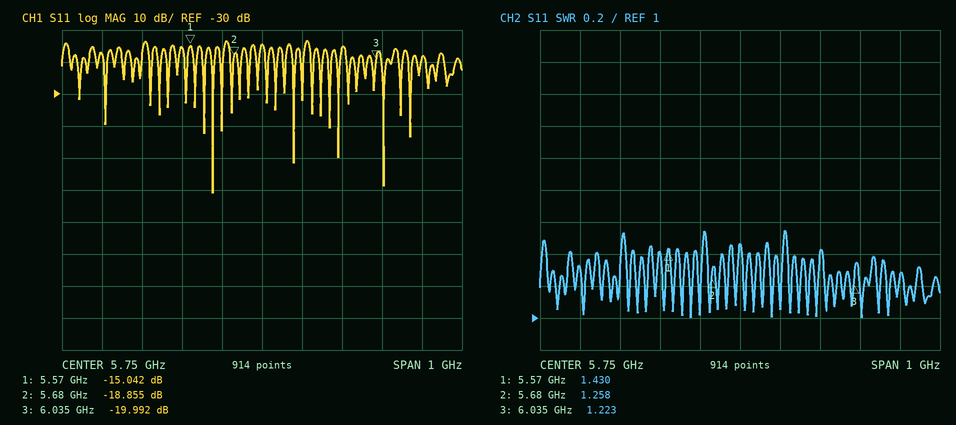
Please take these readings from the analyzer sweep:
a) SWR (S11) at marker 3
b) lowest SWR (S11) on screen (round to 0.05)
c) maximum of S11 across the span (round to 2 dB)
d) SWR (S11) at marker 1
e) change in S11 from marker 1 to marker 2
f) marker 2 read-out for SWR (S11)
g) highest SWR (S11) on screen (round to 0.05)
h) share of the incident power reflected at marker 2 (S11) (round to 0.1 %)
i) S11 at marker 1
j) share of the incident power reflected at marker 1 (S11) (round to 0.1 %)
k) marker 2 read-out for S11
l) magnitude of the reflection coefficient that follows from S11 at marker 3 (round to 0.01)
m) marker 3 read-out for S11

1.223
1.00
-14 dB
1.430
-3.813 dB
1.258
1.55
1.3 %
-15.042 dB
3.1 %
-18.855 dB
0.10
-19.992 dB
